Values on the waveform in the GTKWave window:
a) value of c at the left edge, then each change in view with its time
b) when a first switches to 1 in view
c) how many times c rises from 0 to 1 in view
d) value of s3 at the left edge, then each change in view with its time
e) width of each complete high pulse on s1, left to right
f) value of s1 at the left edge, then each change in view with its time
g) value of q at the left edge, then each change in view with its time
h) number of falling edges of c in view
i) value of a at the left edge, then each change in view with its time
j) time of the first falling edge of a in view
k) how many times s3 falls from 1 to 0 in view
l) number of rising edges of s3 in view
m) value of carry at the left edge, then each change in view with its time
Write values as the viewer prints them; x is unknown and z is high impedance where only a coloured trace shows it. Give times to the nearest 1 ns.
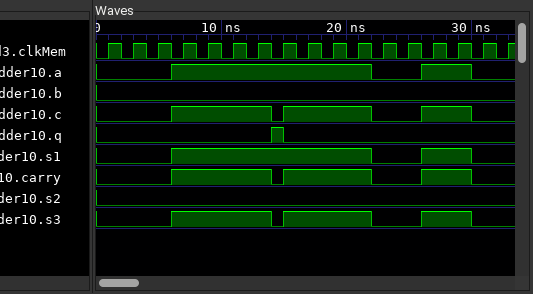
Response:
0, 1 at 6 ns, 0 at 14 ns, 1 at 15 ns, 0 at 22 ns, 1 at 26 ns, 0 at 30 ns
6 ns
3
0, 1 at 6 ns, 0 at 14 ns, 1 at 15 ns, 0 at 22 ns, 1 at 26 ns, 0 at 30 ns
16 ns, 4 ns
0, 1 at 6 ns, 0 at 22 ns, 1 at 26 ns, 0 at 30 ns
0, 1 at 14 ns, 0 at 15 ns
3
0, 1 at 6 ns, 0 at 22 ns, 1 at 26 ns, 0 at 30 ns
22 ns
3
3
0, 1 at 6 ns, 0 at 14 ns, 1 at 15 ns, 0 at 22 ns, 1 at 26 ns, 0 at 30 ns
